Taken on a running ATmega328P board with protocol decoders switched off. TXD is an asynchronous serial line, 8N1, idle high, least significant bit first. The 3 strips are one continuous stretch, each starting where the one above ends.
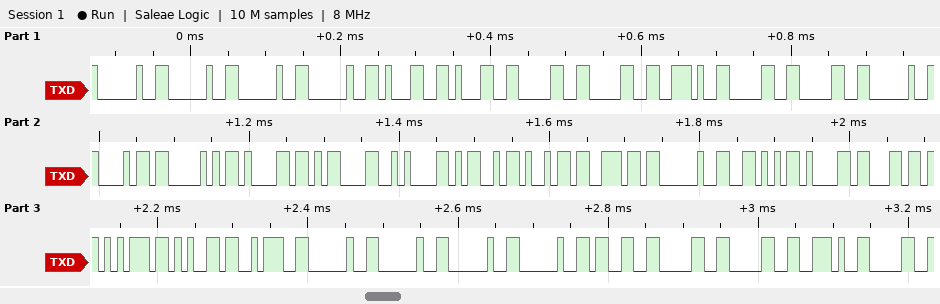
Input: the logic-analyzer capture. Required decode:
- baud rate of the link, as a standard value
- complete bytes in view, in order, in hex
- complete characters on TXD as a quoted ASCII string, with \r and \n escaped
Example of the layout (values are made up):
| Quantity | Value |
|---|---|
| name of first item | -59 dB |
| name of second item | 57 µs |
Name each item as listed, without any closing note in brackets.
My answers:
| Quantity | Value |
|---|---|
| baud rate of the link, as a standard value | 115200 baud |
| complete bytes in view, in order, in hex | 0x20 0x20 0x20 0x20 0x31 0x31 0x30 0x30 0x2E 0x30 0x30 0x20 0x68 0x50 0x61 0x0D 0x0A 0x4D 0x69 0x6E 0x20 0x56 0x61 0x6C 0x75 0x65 0x3A 0x20 0x20 0x20 0x20 0x33 0x30 0x30 0x2E 0x30 |
| complete characters on TXD as a quoted ASCII string, with \r and \n escaped | "    1100.00 hPa\r\nMin Value:    300.0" |
